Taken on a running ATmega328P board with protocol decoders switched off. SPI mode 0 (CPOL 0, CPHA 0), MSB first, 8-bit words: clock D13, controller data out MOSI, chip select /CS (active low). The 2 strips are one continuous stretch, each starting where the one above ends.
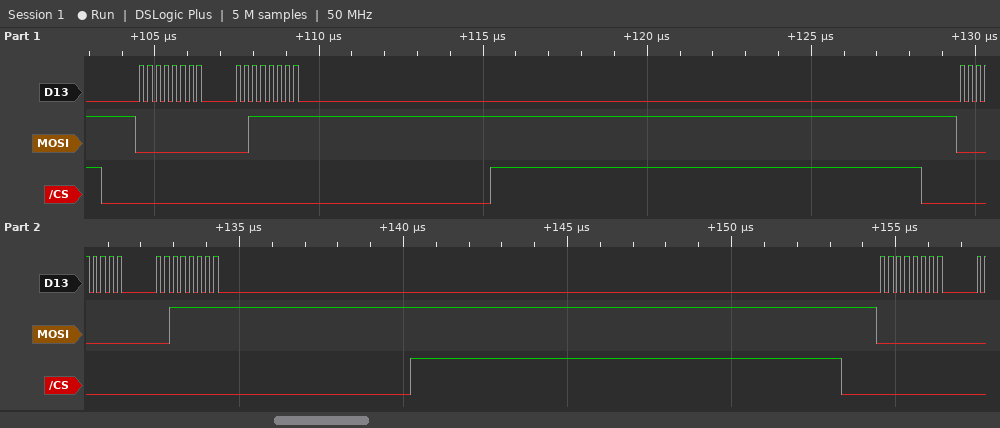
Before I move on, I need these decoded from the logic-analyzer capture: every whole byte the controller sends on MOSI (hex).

00 3F 00 3F 00
